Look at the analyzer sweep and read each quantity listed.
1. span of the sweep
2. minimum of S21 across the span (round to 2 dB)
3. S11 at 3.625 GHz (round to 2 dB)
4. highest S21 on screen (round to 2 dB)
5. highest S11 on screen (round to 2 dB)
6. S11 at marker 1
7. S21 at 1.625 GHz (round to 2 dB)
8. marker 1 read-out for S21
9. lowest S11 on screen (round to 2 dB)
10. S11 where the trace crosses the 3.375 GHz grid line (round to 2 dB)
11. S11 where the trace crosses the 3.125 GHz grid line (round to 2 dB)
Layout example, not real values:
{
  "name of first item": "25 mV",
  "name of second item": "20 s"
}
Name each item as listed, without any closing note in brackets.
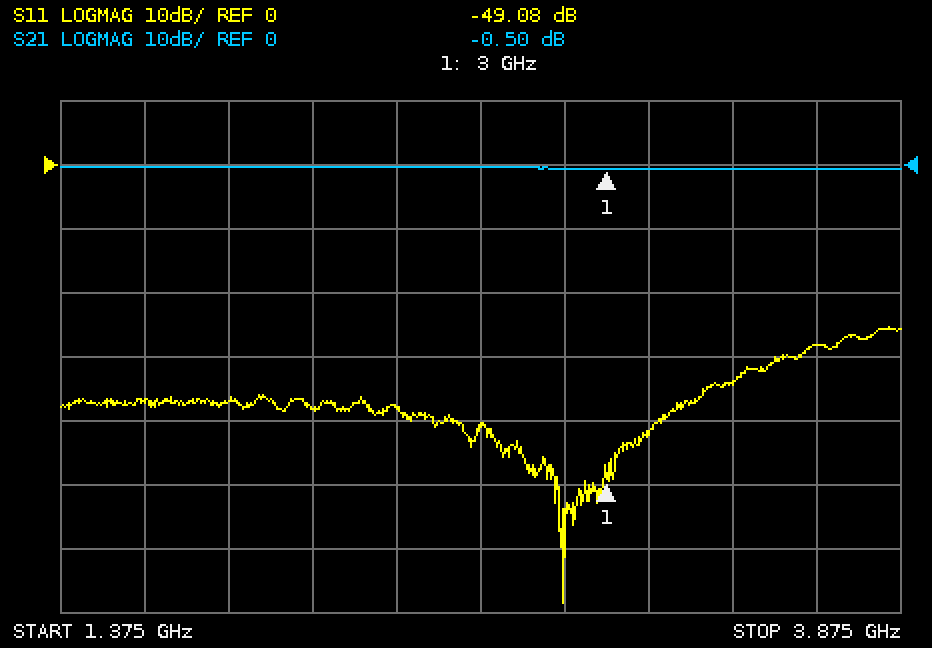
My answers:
{
  "span of the sweep": "2.5 GHz",
  "minimum of S21 across the span": "0 dB",
  "S11 at 3.625 GHz": "-28 dB",
  "highest S21 on screen": "0 dB",
  "highest S11 on screen": "-26 dB",
  "S11 at marker 1": "-49.08 dB",
  "S21 at 1.625 GHz": "0 dB",
  "marker 1 read-out for S21": "-0.50 dB",
  "lowest S11 on screen": "-68 dB",
  "S11 where the trace crosses the 3.375 GHz grid line": "-34 dB",
  "S11 where the trace crosses the 3.125 GHz grid line": "-42 dB"
}
